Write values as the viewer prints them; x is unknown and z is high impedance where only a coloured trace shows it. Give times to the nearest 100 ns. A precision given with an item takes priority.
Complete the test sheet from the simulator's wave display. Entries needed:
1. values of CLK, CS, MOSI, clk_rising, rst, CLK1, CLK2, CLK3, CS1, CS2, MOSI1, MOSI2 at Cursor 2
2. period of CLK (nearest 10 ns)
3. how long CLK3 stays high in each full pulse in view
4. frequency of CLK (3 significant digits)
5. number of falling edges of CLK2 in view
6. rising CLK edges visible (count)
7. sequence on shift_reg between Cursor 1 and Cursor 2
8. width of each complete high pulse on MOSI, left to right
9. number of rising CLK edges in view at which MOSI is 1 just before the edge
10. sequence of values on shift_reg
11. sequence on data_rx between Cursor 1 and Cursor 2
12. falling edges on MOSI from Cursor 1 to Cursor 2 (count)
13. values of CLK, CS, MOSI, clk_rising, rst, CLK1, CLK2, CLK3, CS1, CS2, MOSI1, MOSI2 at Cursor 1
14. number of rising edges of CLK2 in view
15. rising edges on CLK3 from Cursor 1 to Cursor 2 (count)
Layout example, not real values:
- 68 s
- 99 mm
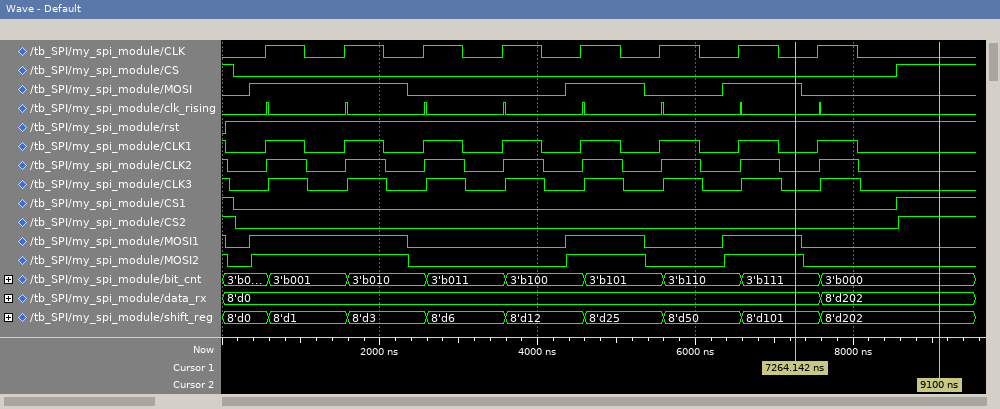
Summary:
- CLK=0, CS=1, MOSI=0, clk_rising=0, rst=1, CLK1=0, CLK2=0, CLK3=0, CS1=1, CS2=1, MOSI1=0, MOSI2=0
- 1000 ns
- 500 ns, 500 ns, 500 ns, 500 ns, 500 ns, 500 ns, 500 ns, 500 ns
- 1.00 MHz
- 9
- 8
- 8'd101, 8'd202
- 2000 ns, 1000 ns, 1000 ns
- 4
- 8'd0, 8'd1, 8'd3, 8'd6, 8'd12, 8'd25, 8'd50, 8'd101, 8'd202
- 8'd0, 8'd202
- 1
- CLK=0, CS=0, MOSI=1, clk_rising=0, rst=1, CLK1=0, CLK2=0, CLK3=0, CS1=0, CS2=0, MOSI1=1, MOSI2=1
- 8
- 1
